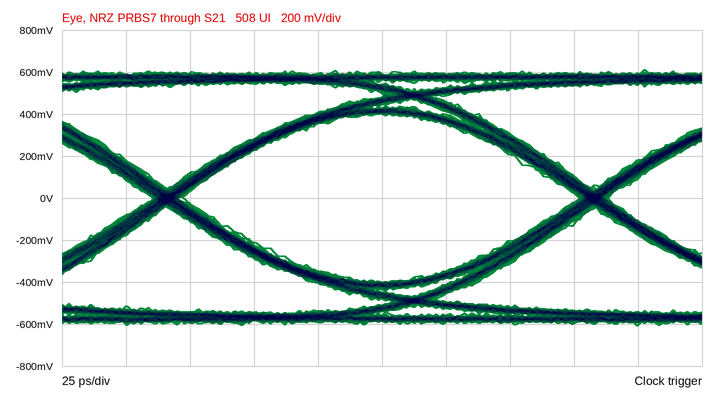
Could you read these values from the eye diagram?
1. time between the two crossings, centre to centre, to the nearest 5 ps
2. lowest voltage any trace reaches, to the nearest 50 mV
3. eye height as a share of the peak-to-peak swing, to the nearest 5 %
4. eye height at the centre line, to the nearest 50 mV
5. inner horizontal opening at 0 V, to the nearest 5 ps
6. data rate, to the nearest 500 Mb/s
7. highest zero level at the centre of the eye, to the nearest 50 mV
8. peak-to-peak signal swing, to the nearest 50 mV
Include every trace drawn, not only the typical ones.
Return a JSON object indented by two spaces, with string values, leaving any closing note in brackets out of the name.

{
  "time between the two crossings, centre to centre, to the nearest 5 ps": "165 ps",
  "lowest voltage any trace reaches, to the nearest 50 mV": "-600 mV",
  "eye height as a share of the peak-to-peak swing, to the nearest 5 %": "65 %",
  "eye height at the centre line, to the nearest 50 mV": "800 mV",
  "inner horizontal opening at 0 V, to the nearest 5 ps": "155 ps",
  "data rate, to the nearest 500 Mb/s": "6.0 Gb/s",
  "highest zero level at the centre of the eye, to the nearest 50 mV": "-400 mV",
  "peak-to-peak signal swing, to the nearest 50 mV": "1.20 V"
}
